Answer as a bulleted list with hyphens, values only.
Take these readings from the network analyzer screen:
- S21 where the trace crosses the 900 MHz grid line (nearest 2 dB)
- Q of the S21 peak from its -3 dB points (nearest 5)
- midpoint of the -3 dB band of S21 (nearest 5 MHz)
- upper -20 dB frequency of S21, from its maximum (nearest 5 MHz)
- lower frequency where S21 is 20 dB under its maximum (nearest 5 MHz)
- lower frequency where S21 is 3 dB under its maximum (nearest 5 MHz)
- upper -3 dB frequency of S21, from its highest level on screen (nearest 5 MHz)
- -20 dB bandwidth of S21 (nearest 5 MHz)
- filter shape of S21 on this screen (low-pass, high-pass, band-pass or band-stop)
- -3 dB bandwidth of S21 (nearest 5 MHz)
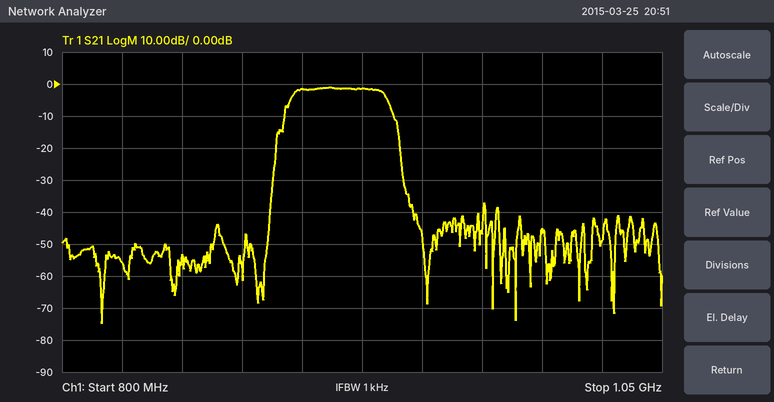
- -2 dB
- 25
- 915 MHz
- 940 MHz
- 890 MHz
- 895 MHz
- 935 MHz
- 50 MHz
- band-pass
- 40 MHz
